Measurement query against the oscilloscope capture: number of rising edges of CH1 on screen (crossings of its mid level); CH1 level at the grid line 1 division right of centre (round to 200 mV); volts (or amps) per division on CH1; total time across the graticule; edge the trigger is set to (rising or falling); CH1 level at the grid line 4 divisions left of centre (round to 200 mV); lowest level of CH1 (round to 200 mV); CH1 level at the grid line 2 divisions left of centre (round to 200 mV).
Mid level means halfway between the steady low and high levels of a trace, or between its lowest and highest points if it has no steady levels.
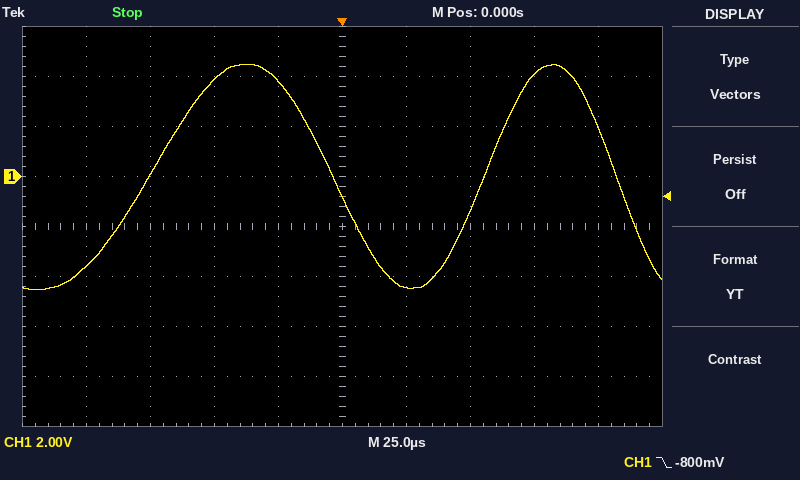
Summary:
2
-4.4 V
2 V
250 µs
falling
-3.6 V
-4.6 V
3.8 V
